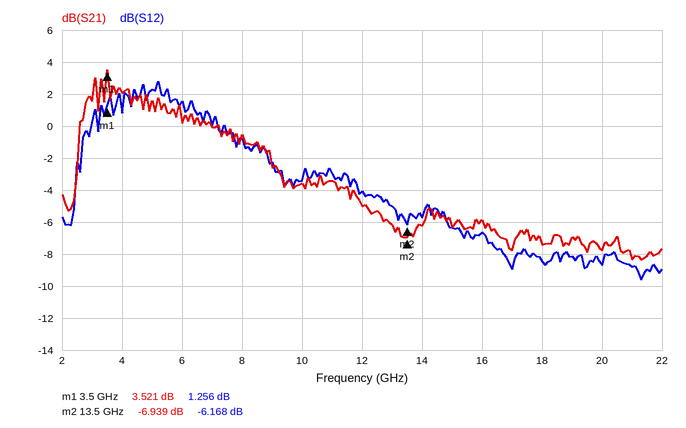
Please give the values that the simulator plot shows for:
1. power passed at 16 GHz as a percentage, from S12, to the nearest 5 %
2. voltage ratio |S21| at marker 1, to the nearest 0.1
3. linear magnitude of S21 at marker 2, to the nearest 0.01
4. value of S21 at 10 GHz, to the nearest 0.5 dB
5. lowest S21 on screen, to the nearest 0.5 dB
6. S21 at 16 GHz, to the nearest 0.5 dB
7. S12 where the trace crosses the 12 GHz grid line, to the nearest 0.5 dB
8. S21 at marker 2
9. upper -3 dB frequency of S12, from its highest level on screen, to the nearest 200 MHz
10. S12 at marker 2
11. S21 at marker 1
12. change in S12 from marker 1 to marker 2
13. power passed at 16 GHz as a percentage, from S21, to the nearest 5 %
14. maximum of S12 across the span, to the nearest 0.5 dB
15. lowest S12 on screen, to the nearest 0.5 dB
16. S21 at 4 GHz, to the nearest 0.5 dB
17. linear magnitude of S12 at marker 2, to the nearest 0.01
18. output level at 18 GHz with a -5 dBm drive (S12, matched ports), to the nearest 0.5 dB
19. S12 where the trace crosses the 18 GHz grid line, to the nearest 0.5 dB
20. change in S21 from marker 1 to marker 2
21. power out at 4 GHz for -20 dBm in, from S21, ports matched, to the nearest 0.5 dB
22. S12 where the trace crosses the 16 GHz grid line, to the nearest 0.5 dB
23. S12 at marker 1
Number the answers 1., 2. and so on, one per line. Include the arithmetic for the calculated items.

1. 10^(-6.5/10) ≈ 22.4 %, so 20 % to the nearest 5 %
2. 10^(3.521/20) ≈ 1.5
3. 10^(-6.939/20) ≈ 0.45
4. -3.5 dB
5. -8.5 dB
6. -6.0 dB
7. -4.0 dB
8. -6.939 dB
9. 7.2 GHz
10. -6.168 dB
11. 3.521 dB
12. -6.168 − (1.256) = -7.424 dB
13. 10^(-6/10) ≈ 25 %
14. 3.0 dB
15. -9.5 dB
16. 2.0 dB
17. 10^(-6.168/20) ≈ 0.49
18. -5 dBm + (-8.5 dB) = -13.5 dBm
19. -8.5 dB
20. -6.939 − (3.521) = -10.460 dB
21. -20 dBm + (2.0 dB) = -18.0 dBm
22. -6.5 dB
23. 1.256 dB
